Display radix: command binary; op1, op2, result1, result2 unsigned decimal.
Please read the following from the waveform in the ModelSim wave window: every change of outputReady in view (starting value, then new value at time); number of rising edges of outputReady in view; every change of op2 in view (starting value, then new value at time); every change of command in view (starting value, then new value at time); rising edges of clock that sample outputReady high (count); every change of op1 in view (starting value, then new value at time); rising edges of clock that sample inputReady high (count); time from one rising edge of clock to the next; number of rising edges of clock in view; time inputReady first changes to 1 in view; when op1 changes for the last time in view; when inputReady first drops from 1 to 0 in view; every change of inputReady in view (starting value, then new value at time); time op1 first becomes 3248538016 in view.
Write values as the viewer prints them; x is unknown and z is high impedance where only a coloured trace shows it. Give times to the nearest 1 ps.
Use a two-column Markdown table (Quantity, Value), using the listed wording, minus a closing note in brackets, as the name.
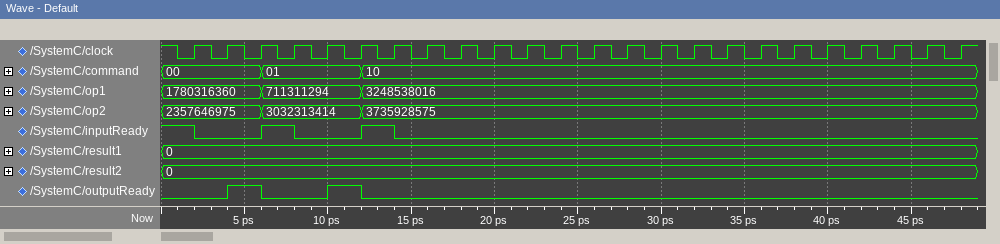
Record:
| Quantity | Value |
|---|---|
| every change of outputReady in view | 0, 1 at 4 ps, 0 at 6 ps, 1 at 10 ps, 0 at 12 ps |
| number of rising edges of outputReady in view | 2 |
| every change of op2 in view | 2357646975, 3032313414 at 6 ps, 3735928575 at 12 ps |
| every change of command in view | 00, 01 at 6 ps, 10 at 12 ps |
| rising edges of clock that sample outputReady high | 2 |
| every change of op1 in view | 1780316360, 711311294 at 6 ps, 3248538016 at 12 ps |
| rising edges of clock that sample inputReady high | 3 |
| time from one rising edge of clock to the next | 2 ps |
| number of rising edges of clock in view | 24 |
| time inputReady first changes to 1 in view | 6 ps |
| when op1 changes for the last time in view | 12 ps |
| when inputReady first drops from 1 to 0 in view | 2 ps |
| every change of inputReady in view | 1, 0 at 2 ps, 1 at 6 ps, 0 at 8 ps, 1 at 12 ps, 0 at 14 ps |
| time op1 first becomes 3248538016 in view | 12 ps |
